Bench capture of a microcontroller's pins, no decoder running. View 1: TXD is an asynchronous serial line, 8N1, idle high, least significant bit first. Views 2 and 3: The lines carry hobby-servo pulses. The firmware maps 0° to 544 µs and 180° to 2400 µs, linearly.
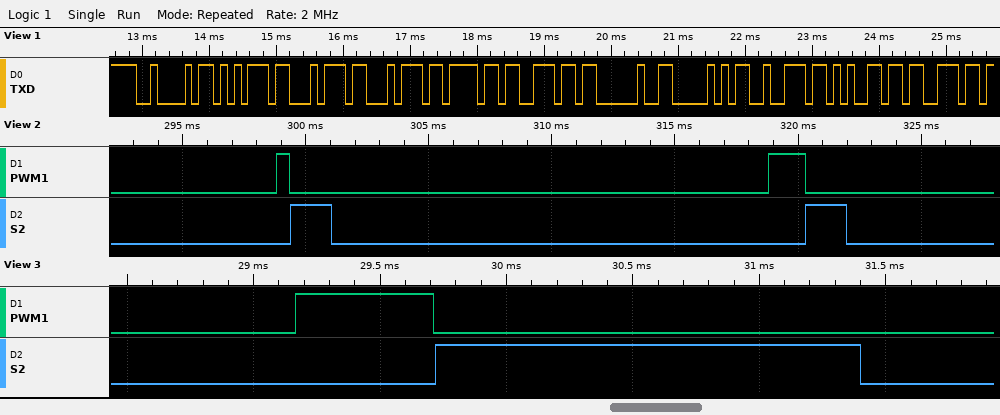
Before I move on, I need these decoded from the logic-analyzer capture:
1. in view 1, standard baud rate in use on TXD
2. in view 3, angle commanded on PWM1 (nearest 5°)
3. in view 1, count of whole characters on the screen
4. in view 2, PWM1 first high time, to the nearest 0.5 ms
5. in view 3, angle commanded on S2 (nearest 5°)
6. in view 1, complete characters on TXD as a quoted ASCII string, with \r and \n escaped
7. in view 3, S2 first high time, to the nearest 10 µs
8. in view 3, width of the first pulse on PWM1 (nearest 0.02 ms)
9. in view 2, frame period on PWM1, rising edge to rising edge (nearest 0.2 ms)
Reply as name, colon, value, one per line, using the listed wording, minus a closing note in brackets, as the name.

in view 1, standard baud rate in use on TXD: 9600 baud
in view 3, angle commanded on PWM1: 0°
in view 1, count of whole characters on the screen: 11
in view 2, PWM1 first high time, to the nearest 0.5 ms: 0.5 ms
in view 3, angle commanded on S2: 110°
in view 1, complete characters on TXD as a quoted ASCII string, with \r and \n escaped: "Button Pres"
in view 3, S2 first high time, to the nearest 10 µs: 1680 µs
in view 3, width of the first pulse on PWM1: 0.54 ms
in view 2, frame period on PWM1, rising edge to rising edge: 20.0 ms
